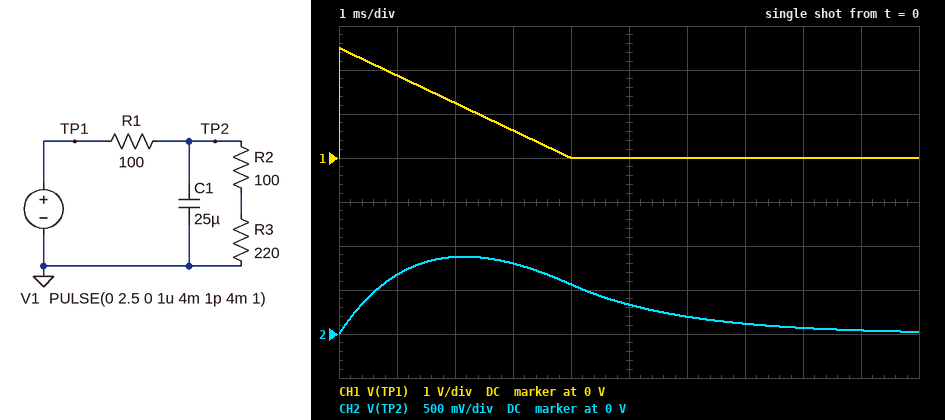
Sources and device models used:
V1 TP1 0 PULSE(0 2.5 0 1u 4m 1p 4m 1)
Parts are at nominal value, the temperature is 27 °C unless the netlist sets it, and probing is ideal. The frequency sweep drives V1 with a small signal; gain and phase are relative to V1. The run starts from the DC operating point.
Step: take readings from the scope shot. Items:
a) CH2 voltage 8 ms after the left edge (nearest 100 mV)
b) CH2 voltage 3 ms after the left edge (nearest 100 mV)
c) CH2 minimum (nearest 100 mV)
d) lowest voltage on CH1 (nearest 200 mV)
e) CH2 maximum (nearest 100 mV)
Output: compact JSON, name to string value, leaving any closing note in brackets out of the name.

{"CH2 voltage 8 ms after the left edge": "100 mV", "CH2 voltage 3 ms after the left edge": "800 mV", "CH2 minimum": "0 V", "lowest voltage on CH1": "0 V", "CH2 maximum": "900 mV"}
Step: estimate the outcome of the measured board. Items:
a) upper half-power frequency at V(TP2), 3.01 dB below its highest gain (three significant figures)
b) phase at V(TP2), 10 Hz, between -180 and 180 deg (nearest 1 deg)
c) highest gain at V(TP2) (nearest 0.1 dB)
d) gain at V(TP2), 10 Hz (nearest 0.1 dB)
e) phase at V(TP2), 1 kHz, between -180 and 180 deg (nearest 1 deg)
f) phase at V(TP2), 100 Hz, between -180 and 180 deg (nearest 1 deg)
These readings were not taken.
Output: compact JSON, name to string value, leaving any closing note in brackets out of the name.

{"upper half-power frequency at V(TP2), 3.01 dB below its highest gain": "83.6 Hz", "phase at V(TP2), 10 Hz, between -180 and 180 deg": "-7 deg", "highest gain at V(TP2)": "-2.4 dB", "gain at V(TP2), 10 Hz": "-2.4 dB", "phase at V(TP2), 1 kHz, between -180 and 180 deg": "-85 deg", "phase at V(TP2), 100 Hz, between -180 and 180 deg": "-50 deg"}
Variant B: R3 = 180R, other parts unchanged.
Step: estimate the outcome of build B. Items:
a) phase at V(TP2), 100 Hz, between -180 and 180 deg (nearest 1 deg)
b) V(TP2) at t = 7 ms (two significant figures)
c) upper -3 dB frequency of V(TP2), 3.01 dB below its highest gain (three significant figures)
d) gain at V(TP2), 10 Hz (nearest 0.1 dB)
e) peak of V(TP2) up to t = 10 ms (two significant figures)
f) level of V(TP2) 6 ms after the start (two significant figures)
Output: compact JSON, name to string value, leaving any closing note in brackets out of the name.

{"phase at V(TP2), 100 Hz, between -180 and 180 deg": "-49 deg", "V(TP2) at t = 7 ms": "110 mV", "upper -3 dB frequency of V(TP2), 3.01 dB below its highest gain": "86.4 Hz", "gain at V(TP2), 10 Hz": "-2.7 dB", "peak of V(TP2) up to t = 10 ms": "860 mV", "level of V(TP2) 6 ms after the start": "180 mV"}
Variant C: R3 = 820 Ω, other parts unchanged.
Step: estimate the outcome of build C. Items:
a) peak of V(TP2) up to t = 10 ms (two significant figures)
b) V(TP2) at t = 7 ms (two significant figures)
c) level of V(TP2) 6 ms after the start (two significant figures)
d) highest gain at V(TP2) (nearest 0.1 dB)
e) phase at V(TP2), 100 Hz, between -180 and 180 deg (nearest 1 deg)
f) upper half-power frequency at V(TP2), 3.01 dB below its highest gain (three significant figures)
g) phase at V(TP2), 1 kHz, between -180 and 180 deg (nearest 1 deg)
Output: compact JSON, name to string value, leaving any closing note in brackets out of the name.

{"peak of V(TP2) up to t = 10 ms": "960 mV", "V(TP2) at t = 7 ms": "180 mV", "level of V(TP2) 6 ms after the start": "280 mV", "highest gain at V(TP2)": "-0.9 dB", "phase at V(TP2), 100 Hz, between -180 and 180 deg": "-55 deg", "upper half-power frequency at V(TP2), 3.01 dB below its highest gain": "70.6 Hz", "phase at V(TP2), 1 kHz, between -180 and 180 deg": "-86 deg"}
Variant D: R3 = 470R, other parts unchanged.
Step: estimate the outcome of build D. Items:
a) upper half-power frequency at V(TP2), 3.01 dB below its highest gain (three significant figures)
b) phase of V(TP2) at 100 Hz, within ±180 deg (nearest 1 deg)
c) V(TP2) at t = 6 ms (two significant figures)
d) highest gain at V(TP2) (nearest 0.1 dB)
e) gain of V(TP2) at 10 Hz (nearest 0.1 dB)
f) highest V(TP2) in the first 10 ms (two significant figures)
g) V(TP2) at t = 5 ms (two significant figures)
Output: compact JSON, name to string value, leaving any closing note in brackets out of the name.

{"upper half-power frequency at V(TP2), 3.01 dB below its highest gain": "74.8 Hz", "phase of V(TP2) at 100 Hz, within ±180 deg": "-53 deg", "V(TP2) at t = 6 ms": "250 mV", "highest gain at V(TP2)": "-1.4 dB", "gain of V(TP2) at 10 Hz": "-1.5 dB", "highest V(TP2) in the first 10 ms": "930 mV", "V(TP2) at t = 5 ms": "400 mV"}
